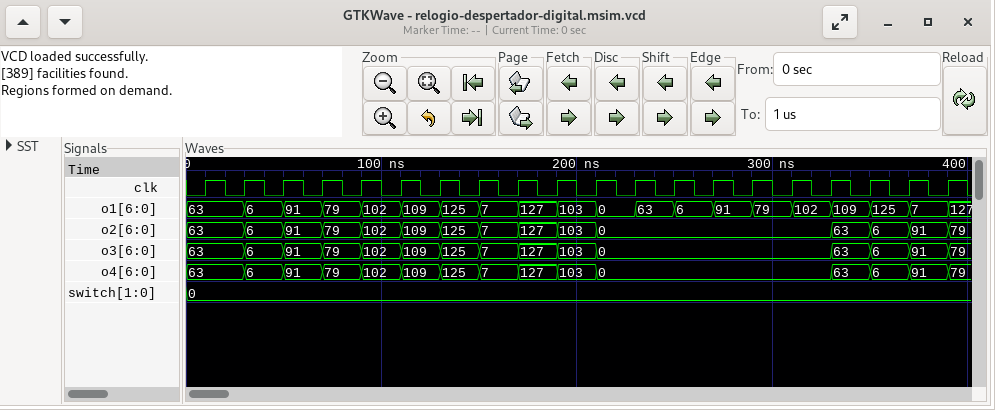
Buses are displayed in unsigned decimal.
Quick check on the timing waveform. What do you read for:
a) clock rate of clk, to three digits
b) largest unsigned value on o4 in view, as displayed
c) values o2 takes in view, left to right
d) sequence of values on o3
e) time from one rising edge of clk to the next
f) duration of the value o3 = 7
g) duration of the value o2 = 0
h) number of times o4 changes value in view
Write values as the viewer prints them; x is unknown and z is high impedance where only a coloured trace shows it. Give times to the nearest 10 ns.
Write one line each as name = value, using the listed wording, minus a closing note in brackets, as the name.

clock rate of clk, to three digits = 50.0 MHz
largest unsigned value on o4 in view, as displayed = 127
values o2 takes in view, left to right = 63, 6, 91, 79, 102, 109, 125, 7, 127, 103, 0, 63, 6, 91, 79
sequence of values on o3 = 63, 6, 91, 79, 102, 109, 125, 7, 127, 103, 0, 63, 6, 91, 79
time from one rising edge of clk to the next = 20 ns
duration of the value o3 = 7 = 20 ns
duration of the value o2 = 0 = 120 ns
number of times o4 changes value in view = 14
